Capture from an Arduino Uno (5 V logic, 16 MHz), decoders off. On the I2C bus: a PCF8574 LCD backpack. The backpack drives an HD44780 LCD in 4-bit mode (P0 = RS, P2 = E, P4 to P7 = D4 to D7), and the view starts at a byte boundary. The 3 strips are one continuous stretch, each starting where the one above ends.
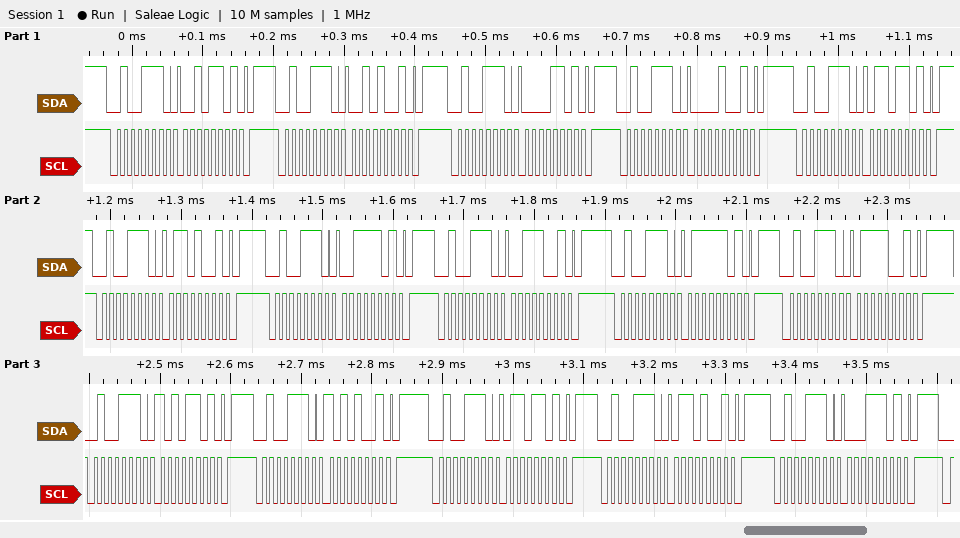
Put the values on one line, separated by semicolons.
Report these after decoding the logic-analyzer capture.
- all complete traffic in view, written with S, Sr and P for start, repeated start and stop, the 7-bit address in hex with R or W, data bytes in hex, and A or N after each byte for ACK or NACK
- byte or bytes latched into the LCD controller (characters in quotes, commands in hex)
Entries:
S 27W A 2D A P S 27W A 29 A P S 27W A 0D A P S 27W A 09 A P S 27W A 6D A P S 27W A 69 A P S 27W A 3D A P S 27W A 39 A P S 27W A 7D A P S 27W A 79 A P S 27W A AD A P S 27W A A9 A P S 27W A 6D A P S 27W A 69 A P S 27W A 1D A P; ' ' 'c' 'z'
